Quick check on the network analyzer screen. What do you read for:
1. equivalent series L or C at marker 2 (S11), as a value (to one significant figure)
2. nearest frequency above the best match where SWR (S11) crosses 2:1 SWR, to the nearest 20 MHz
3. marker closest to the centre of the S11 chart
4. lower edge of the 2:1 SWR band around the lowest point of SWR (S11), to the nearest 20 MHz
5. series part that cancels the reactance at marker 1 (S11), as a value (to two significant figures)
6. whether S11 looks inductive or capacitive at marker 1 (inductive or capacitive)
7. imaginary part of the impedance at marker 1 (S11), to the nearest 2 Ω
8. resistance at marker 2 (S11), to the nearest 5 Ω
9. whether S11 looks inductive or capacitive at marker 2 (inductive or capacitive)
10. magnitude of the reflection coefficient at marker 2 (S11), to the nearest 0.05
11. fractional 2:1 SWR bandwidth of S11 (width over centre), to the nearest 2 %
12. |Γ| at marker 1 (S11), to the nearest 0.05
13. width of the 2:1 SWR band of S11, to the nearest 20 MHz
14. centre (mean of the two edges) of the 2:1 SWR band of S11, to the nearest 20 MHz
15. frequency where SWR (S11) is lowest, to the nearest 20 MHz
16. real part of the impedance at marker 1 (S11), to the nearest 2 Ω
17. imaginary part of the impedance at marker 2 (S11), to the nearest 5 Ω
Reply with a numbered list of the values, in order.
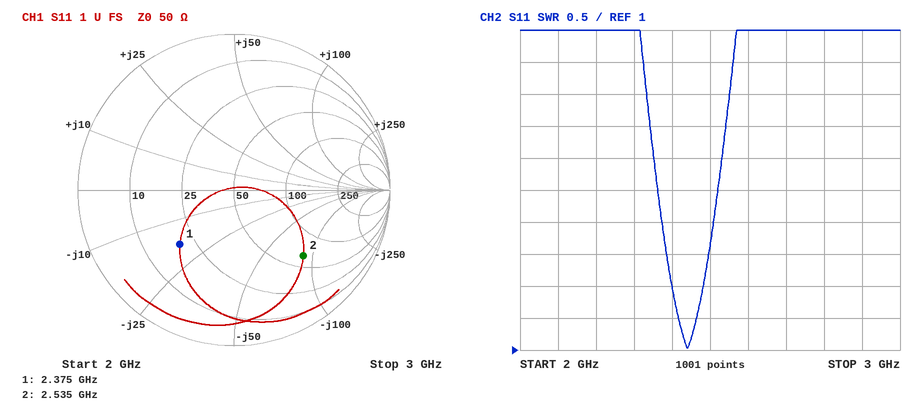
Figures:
1. 700 fF
2. 2.48 GHz
3. marker 1
4. 2.40 GHz
5. 1.2 nH
6. capacitive
7. -18 Ω
8. 65 Ω
9. capacitive
10. 0.60
11. 4 %
12. 0.50
13. 80 MHz
14. 2.44 GHz
15. 2.44 GHz
16. 20 Ω
17. -85 Ω
